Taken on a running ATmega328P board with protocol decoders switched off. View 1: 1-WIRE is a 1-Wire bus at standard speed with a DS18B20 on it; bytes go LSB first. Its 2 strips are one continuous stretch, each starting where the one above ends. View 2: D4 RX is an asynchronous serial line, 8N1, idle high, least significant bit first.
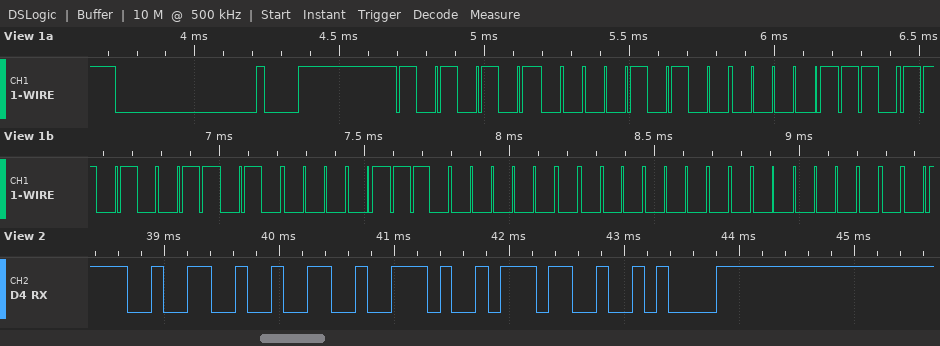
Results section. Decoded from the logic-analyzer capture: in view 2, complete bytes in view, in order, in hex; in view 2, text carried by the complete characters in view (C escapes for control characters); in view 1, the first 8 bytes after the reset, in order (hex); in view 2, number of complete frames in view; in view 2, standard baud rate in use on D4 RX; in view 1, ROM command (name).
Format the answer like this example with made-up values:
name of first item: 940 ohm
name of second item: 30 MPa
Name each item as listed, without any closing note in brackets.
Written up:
in view 2, complete bytes in view, in order, in hex: 32 32 2E 37 0A
in view 2, text carried by the complete characters in view: "22.7\n"
in view 1, the first 8 bytes after the reset, in order: 55 28 70 CB 82 03 00 00
in view 2, number of complete frames in view: 5
in view 2, standard baud rate in use on D4 RX: 9600 baud
in view 1, ROM command: Match ROM
